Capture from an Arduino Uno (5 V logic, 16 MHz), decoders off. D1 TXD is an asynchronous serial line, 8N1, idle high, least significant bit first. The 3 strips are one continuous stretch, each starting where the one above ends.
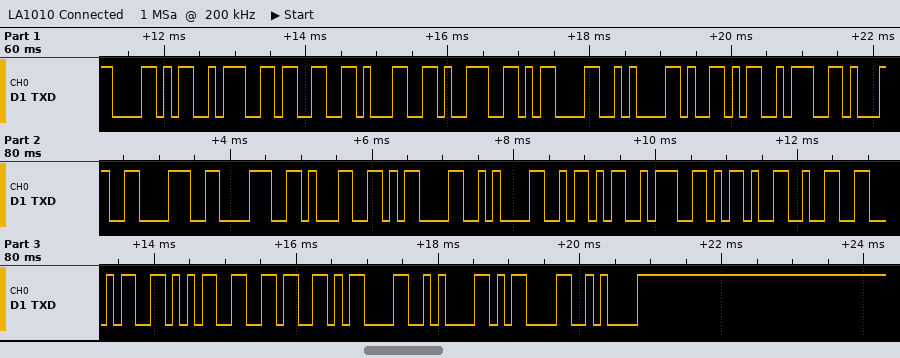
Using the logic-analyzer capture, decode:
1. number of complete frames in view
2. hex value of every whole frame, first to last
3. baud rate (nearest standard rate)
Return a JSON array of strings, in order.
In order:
["26", "0x58 0x3A 0x33 0x31 0x39 0x0D 0x0A 0x59 0x3A 0x31 0x38 0x38 0x31 0x0D 0x0A 0x5A 0x3A 0x2D 0x32 0x34 0x35 0x36 0x0D 0x0A 0x0D 0x0A", "9600 baud"]
